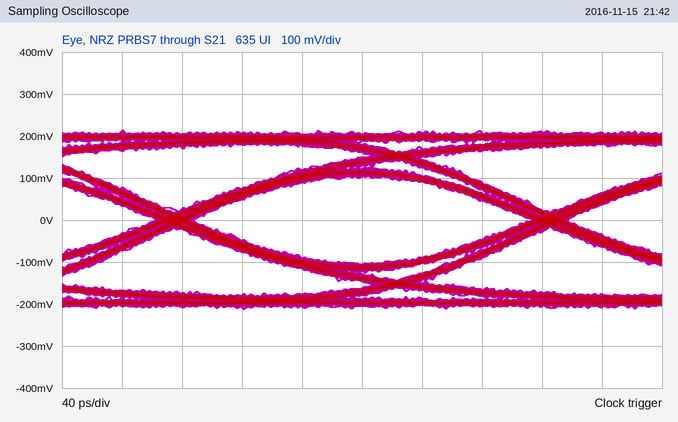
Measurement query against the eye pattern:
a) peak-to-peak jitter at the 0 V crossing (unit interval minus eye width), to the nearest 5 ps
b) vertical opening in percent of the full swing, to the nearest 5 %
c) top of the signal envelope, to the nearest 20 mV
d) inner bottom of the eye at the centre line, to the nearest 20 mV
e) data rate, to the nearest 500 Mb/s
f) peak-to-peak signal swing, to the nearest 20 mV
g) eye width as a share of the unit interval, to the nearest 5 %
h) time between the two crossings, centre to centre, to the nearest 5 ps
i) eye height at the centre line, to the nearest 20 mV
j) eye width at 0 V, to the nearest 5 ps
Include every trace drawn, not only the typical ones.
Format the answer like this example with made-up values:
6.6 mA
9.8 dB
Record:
25 ps
50 %
220 mV
-100 mV
4.0 Gb/s
420 mV
90 %
250 ps
200 mV
225 ps
